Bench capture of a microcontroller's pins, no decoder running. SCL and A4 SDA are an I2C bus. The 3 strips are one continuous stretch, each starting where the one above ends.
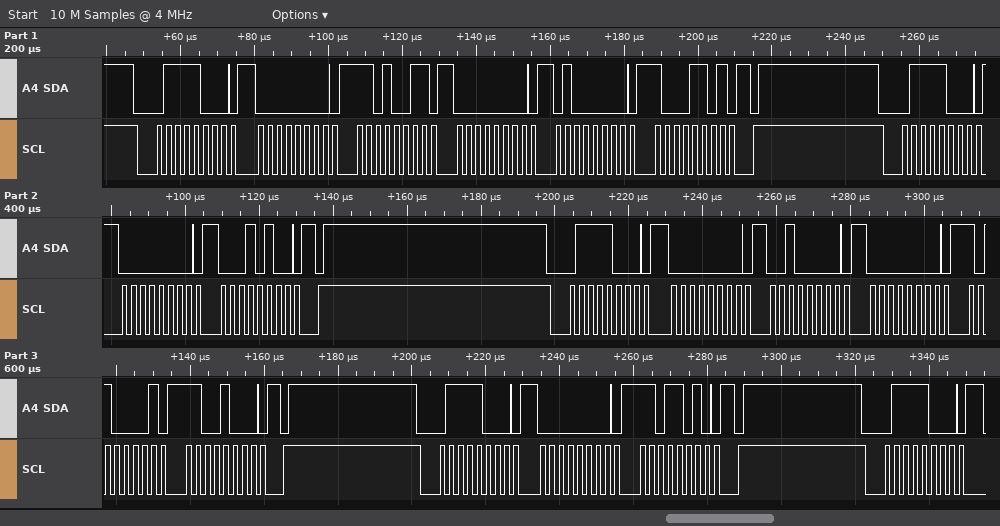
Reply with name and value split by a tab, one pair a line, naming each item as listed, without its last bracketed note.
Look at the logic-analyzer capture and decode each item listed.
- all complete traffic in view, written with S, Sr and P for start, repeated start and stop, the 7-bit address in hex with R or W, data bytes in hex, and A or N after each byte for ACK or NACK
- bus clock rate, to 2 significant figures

all complete traffic in view, written with S, Sr and P for start, repeated start and stop, the 7-bit address in hex with R or W, data bytes in hex, and A or N after each byte for ACK or NACK	S 3CW A 00 A D3 A 00 A 40 A 8D A P S 3CW A 00 A 14 A P S 3CW A 00 A 20 A 00 A A1 A C8 A P S 3CW A 00 A DA A P S 3CW A
bus clock rate, to 2 significant figures	400 kHz
